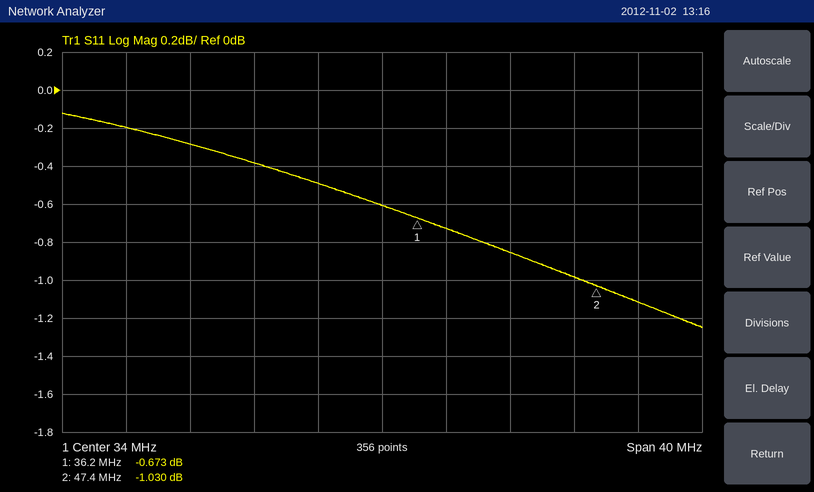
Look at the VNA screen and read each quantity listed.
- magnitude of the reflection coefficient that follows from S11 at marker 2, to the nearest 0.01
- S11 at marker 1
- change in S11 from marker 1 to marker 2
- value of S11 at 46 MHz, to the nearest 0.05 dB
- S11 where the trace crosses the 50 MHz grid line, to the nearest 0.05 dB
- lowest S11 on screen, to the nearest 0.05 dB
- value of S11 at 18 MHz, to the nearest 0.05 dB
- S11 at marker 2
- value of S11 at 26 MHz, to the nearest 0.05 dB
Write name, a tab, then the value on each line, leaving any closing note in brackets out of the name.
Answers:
magnitude of the reflection coefficient that follows from S11 at marker 2, to the nearest 0.01	0.89
S11 at marker 1	-0.673 dB
change in S11 from marker 1 to marker 2	-0.357 dB
value of S11 at 46 MHz, to the nearest 0.05 dB	-1.00 dB
S11 where the trace crosses the 50 MHz grid line, to the nearest 0.05 dB	-1.10 dB
lowest S11 on screen, to the nearest 0.05 dB	-1.25 dB
value of S11 at 18 MHz, to the nearest 0.05 dB	-0.20 dB
S11 at marker 2	-1.030 dB
value of S11 at 26 MHz, to the nearest 0.05 dB	-0.40 dB
